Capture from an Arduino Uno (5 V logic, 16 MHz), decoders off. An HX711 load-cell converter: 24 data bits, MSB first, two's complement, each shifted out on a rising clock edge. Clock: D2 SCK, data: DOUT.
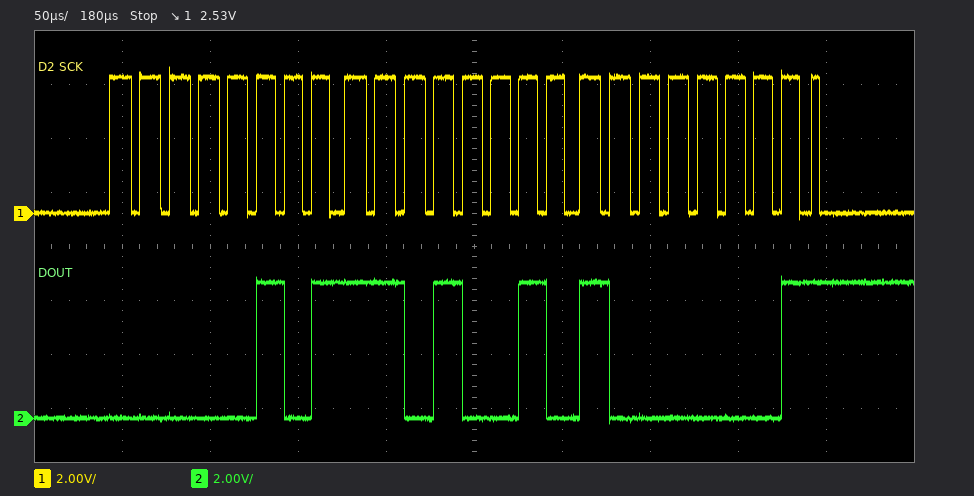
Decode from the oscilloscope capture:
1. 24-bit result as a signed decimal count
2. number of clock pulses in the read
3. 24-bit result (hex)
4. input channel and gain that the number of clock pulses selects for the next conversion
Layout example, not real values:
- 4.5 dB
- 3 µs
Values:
- 381569
- 25
- 0x05D281
- channel A, gain 128
